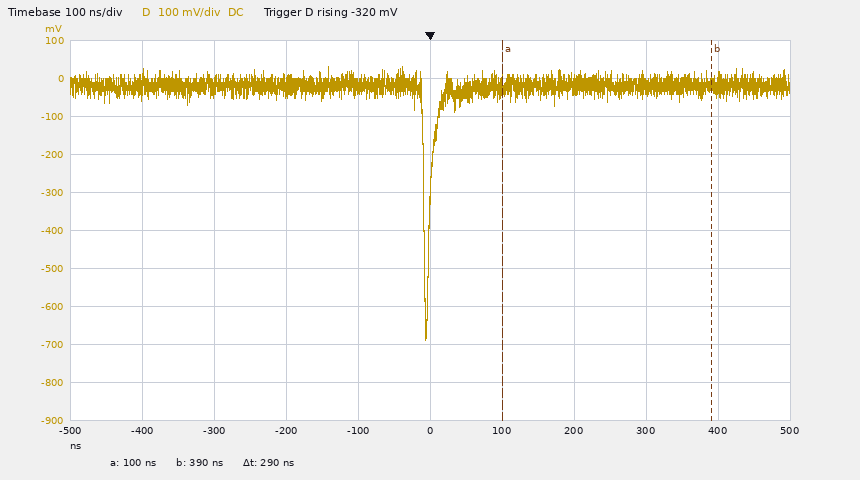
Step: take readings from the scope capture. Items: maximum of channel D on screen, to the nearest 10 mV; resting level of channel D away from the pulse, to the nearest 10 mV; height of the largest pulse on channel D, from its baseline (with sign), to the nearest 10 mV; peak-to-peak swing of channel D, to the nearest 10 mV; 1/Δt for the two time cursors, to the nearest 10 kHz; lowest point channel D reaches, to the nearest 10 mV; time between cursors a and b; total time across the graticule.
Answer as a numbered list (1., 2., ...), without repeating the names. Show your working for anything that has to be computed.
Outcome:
1. 30 mV
2. -20 mV
3. -690 mV − (-20 mV) = -670 mV
4. 30 mV − (-690 mV) = 720 mV
5. 1 / 290 ns ≈ 3.45 MHz
6. -690 mV
7. 290 ns
8. 1 µs
